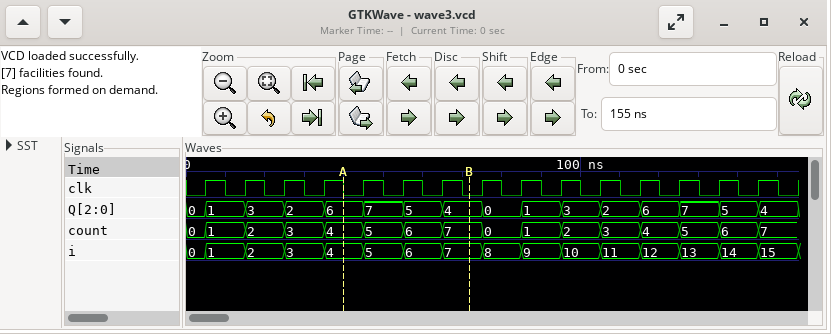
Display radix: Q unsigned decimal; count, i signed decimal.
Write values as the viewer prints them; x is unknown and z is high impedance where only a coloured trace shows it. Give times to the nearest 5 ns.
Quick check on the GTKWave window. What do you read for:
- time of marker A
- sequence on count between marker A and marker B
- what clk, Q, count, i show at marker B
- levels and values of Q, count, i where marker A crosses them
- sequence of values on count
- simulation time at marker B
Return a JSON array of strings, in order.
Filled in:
["40 ns", "4, 5, 6, 7", "clk=0, Q=4, count=7, i=7", "Q=6, count=4, i=4", "0, 1, 2, 3, 4, 5, 6, 7, 0, 1, 2, 3, 4, 5, 6, 7", "70 ns"]
